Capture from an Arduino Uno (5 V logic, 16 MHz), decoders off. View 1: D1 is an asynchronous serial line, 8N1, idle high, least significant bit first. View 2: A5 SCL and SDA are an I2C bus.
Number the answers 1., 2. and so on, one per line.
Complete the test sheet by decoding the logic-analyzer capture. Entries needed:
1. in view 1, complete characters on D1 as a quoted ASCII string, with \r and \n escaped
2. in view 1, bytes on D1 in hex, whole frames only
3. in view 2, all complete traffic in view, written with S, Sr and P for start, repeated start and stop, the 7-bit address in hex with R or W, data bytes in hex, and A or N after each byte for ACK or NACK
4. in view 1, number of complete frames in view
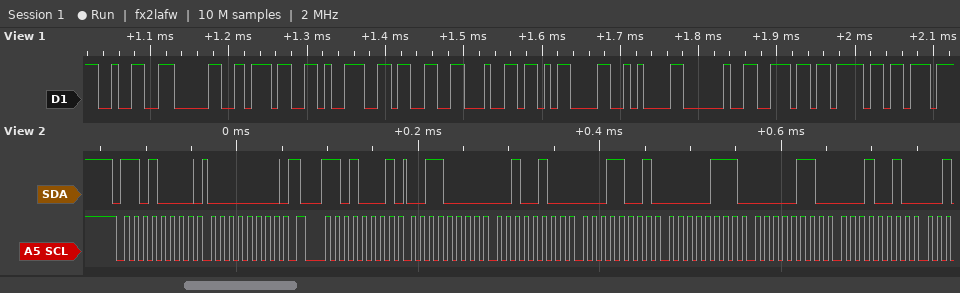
1. "20793d\r\n no"
2. 32 30 37 39 33 64 0D 0A 20 6E 6F
3. S 68W A 00 A Sr 68R A 30 A 24 A 19 A 07 A 06 A 12 A
4. 11
